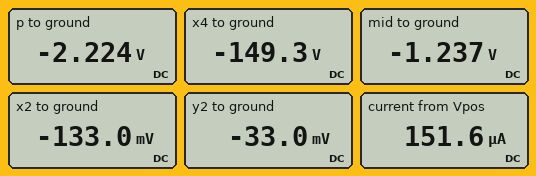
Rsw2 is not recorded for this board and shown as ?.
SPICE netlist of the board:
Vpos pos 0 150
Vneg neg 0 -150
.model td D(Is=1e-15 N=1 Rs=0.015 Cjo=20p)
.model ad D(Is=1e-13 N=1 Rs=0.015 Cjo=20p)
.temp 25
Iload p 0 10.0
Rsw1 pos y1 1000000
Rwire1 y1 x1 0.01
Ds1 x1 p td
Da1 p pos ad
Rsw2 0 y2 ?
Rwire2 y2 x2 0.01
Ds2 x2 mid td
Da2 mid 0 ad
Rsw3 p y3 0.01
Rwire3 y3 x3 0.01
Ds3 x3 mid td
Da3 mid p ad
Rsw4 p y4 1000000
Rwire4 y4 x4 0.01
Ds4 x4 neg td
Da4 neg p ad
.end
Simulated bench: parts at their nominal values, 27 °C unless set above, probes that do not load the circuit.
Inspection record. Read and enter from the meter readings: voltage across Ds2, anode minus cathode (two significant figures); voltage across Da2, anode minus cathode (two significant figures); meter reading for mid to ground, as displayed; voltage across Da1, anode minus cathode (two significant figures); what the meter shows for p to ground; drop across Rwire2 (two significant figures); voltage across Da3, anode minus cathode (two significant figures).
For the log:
1.1 V
-1.2 V
-1.237 V
-150 V
-2.224 V
100 mV
990 mV
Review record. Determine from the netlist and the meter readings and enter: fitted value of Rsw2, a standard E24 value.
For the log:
3.3 mΩ
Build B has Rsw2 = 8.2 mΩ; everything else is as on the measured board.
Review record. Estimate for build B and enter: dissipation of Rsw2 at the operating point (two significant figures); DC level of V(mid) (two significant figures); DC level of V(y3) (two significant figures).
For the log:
820 mW
-1.3 V
-2.3 V
